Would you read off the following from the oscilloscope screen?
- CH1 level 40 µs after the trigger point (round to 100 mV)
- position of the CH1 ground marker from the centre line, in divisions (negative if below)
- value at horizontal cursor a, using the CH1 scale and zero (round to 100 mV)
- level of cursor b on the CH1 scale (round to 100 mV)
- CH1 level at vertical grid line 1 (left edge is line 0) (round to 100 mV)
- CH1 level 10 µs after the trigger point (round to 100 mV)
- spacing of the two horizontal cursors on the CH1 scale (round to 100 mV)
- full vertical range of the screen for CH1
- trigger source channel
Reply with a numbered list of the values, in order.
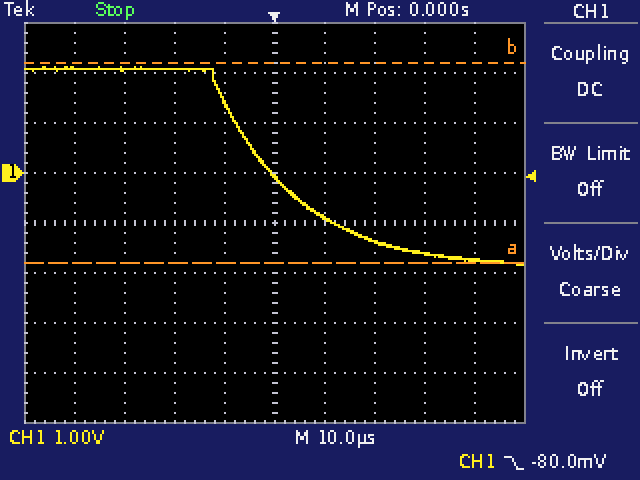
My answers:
1. -1.7 V
2. +1.0 div
3. -1.8 V
4. 2.2 V
5. 2.1 V
6. -900 mV
7. 4.0 V
8. 8 V
9. CH1
